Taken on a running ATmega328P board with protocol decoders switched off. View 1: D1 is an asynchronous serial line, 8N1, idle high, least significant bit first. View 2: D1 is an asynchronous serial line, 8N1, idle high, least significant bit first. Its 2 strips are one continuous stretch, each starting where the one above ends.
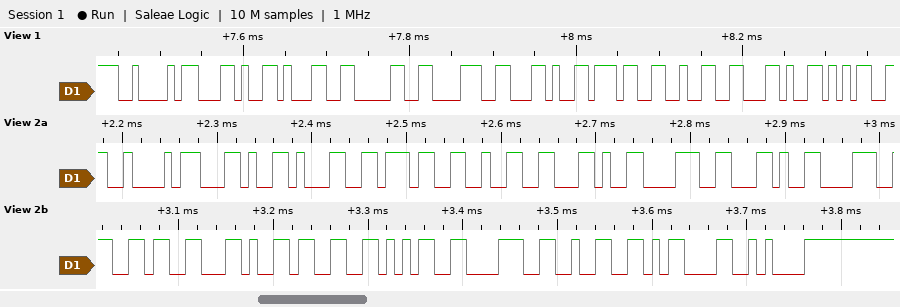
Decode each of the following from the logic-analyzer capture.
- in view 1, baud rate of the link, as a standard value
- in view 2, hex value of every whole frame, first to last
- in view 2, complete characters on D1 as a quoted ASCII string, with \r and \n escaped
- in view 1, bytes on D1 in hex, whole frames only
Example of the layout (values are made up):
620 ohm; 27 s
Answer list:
115200 baud; 42 2C 31 37 32 2C 38 2C 38 36 2C 33 35 38 32 0D 0A; "B,172,8,86,3582\r\n"; 0x42 0x2C 0x31 0x30 0x38 0x2C 0x37 0x32 0x2C 0x35
